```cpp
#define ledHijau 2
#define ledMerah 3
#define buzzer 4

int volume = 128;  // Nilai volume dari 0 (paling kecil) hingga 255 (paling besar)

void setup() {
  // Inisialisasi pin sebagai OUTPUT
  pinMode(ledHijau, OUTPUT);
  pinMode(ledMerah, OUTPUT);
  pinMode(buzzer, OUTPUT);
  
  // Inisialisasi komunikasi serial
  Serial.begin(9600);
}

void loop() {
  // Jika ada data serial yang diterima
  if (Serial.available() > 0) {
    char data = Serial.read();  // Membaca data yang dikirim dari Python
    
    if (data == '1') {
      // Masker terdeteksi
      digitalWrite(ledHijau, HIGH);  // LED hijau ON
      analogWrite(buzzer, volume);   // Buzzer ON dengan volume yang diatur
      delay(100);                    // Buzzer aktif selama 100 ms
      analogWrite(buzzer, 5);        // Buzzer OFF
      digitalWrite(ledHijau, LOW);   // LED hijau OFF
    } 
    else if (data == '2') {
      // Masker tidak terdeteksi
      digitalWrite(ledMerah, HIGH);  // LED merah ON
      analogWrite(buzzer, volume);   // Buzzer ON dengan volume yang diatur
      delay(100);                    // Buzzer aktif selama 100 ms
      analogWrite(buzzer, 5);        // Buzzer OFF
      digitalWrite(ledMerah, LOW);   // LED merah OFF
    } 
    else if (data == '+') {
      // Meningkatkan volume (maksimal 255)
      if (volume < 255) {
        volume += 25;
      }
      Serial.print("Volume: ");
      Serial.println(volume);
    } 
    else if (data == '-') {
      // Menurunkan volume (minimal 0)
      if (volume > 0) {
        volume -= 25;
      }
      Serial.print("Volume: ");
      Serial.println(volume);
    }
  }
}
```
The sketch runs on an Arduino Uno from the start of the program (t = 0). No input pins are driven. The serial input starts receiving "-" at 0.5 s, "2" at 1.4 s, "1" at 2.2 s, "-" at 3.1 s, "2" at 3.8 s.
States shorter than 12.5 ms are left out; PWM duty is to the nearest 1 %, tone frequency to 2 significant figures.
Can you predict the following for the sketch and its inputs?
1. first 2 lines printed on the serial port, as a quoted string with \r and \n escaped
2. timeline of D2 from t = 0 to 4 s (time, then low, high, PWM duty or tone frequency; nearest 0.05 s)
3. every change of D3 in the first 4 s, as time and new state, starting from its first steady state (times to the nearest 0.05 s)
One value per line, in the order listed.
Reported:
"Volume: 103\r\nVolume: 78\r\n"
0 s low; 2.2 s high; 2.3 s low
0 s low; 1.4 s high; 1.5 s low; 3.8 s high; 3.9 s low
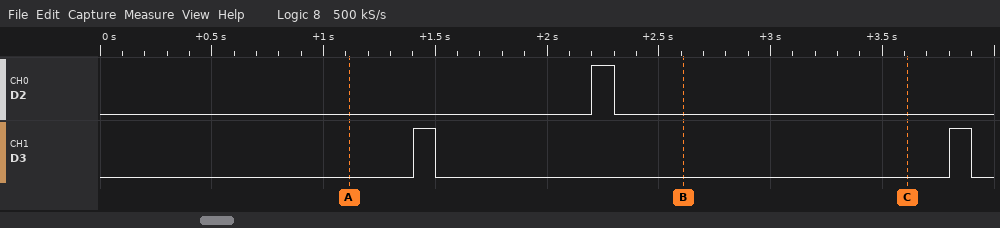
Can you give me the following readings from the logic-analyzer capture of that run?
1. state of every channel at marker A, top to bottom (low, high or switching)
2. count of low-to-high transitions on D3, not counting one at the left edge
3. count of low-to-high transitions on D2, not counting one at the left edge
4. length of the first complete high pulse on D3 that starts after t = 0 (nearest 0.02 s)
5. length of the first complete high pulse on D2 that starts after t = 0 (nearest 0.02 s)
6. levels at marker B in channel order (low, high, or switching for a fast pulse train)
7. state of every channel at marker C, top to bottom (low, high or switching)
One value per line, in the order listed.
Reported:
D2 low, D3 low
2
1
0.10 s
0.10 s
D2 low, D3 low
D2 low, D3 low
